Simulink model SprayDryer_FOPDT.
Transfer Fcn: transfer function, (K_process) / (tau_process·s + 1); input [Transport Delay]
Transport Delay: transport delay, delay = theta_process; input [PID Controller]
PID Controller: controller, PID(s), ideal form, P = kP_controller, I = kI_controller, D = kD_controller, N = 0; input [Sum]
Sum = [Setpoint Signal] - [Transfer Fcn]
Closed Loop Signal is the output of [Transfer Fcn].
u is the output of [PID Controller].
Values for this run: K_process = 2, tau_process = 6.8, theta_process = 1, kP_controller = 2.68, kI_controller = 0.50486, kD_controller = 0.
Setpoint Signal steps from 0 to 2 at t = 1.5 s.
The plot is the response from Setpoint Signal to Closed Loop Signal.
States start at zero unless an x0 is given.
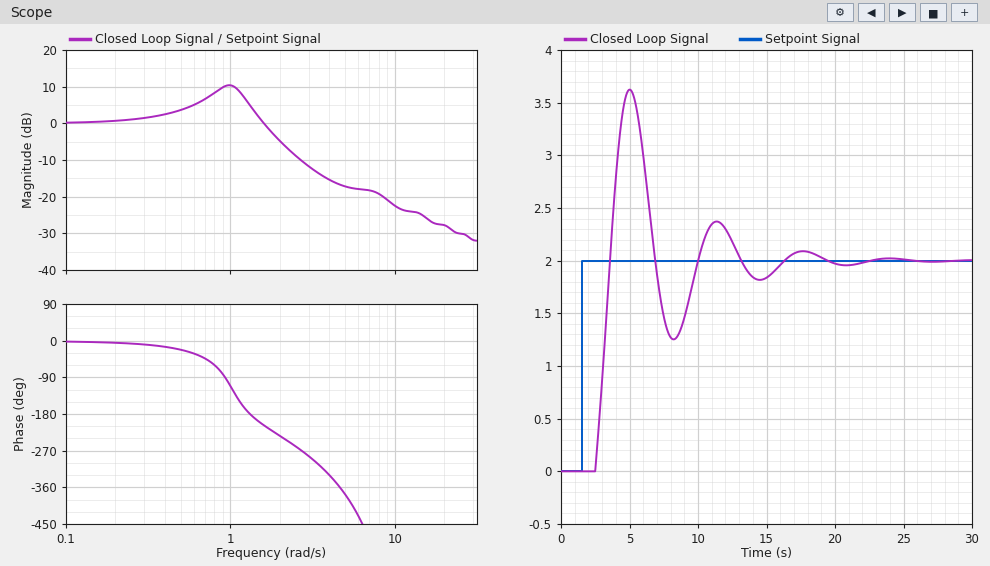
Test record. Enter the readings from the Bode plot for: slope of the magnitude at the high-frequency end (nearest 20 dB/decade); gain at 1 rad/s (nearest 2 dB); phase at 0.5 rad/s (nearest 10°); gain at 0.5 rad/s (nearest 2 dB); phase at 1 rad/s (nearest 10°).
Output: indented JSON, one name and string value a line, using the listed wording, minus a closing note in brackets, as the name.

{
  "slope of the magnitude at the high-frequency end": "-20 dB/decade",
  "gain at 1 rad/s": "10 dB",
  "phase at 0.5 rad/s": "-20°",
  "gain at 0.5 rad/s": "4 dB",
  "phase at 1 rad/s": "-110°"
}
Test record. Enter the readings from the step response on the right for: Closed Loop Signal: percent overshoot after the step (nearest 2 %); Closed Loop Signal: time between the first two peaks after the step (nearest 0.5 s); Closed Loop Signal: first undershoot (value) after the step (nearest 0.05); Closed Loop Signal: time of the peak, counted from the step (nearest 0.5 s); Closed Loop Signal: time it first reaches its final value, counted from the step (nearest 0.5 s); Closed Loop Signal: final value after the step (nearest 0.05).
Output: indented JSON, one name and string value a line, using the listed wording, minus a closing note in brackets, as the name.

{
  "Closed Loop Signal: percent overshoot after the step": "82 %",
  "Closed Loop Signal: time between the first two peaks after the step": "6.5 s",
  "Closed Loop Signal: first undershoot (value) after the step": "1.25",
  "Closed Loop Signal: time of the peak, counted from the step": "3.5 s",
  "Closed Loop Signal: time it first reaches its final value, counted from the step": "2.0 s",
  "Closed Loop Signal: final value after the step": "2.00"
}
